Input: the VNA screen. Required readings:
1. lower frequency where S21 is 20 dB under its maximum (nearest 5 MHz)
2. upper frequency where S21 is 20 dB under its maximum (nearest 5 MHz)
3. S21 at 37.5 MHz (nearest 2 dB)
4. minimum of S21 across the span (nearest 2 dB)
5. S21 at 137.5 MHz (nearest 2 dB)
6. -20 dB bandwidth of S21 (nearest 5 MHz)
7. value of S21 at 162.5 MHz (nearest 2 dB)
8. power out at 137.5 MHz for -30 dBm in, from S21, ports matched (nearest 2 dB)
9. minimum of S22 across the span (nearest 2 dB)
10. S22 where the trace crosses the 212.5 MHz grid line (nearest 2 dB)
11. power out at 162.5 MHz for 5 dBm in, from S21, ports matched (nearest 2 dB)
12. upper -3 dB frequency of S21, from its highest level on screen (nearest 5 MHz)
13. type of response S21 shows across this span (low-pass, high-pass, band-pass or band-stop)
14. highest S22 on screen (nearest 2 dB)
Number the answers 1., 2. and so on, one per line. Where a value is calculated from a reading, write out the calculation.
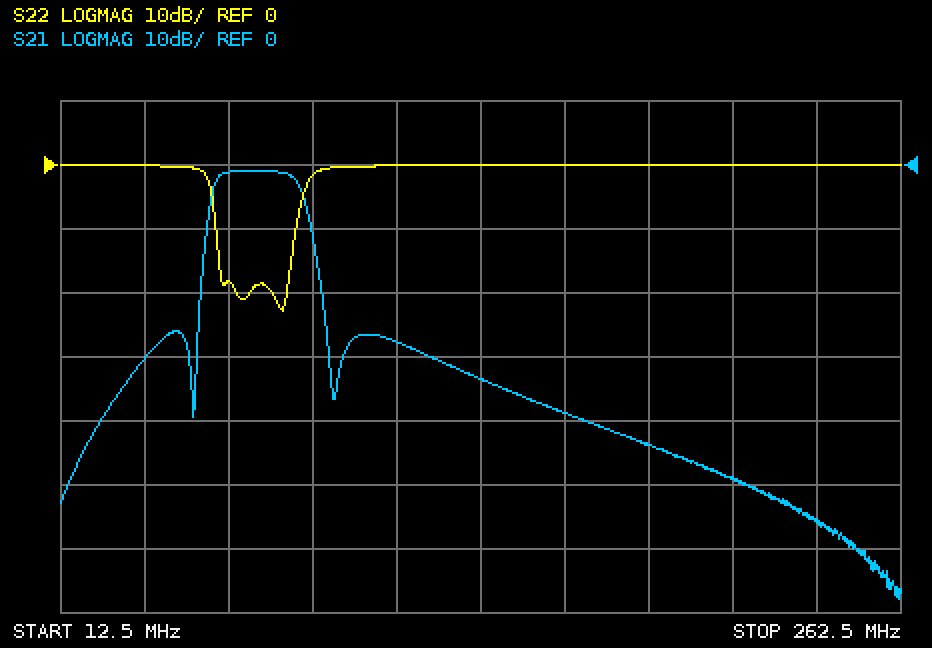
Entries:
1. 55 MHz
2. 90 MHz
3. -30 dB
4. -68 dB
5. -34 dB
6. 90 MHz − 55 MHz = 35 MHz
7. -38 dB
8. -30 dBm + (-34 dB) = -64 dBm
9. -22 dB
10. 0 dB
11. 5 dBm + (-38 dB) = -34 dBm
12. 85 MHz
13. band-pass
14. 0 dB
